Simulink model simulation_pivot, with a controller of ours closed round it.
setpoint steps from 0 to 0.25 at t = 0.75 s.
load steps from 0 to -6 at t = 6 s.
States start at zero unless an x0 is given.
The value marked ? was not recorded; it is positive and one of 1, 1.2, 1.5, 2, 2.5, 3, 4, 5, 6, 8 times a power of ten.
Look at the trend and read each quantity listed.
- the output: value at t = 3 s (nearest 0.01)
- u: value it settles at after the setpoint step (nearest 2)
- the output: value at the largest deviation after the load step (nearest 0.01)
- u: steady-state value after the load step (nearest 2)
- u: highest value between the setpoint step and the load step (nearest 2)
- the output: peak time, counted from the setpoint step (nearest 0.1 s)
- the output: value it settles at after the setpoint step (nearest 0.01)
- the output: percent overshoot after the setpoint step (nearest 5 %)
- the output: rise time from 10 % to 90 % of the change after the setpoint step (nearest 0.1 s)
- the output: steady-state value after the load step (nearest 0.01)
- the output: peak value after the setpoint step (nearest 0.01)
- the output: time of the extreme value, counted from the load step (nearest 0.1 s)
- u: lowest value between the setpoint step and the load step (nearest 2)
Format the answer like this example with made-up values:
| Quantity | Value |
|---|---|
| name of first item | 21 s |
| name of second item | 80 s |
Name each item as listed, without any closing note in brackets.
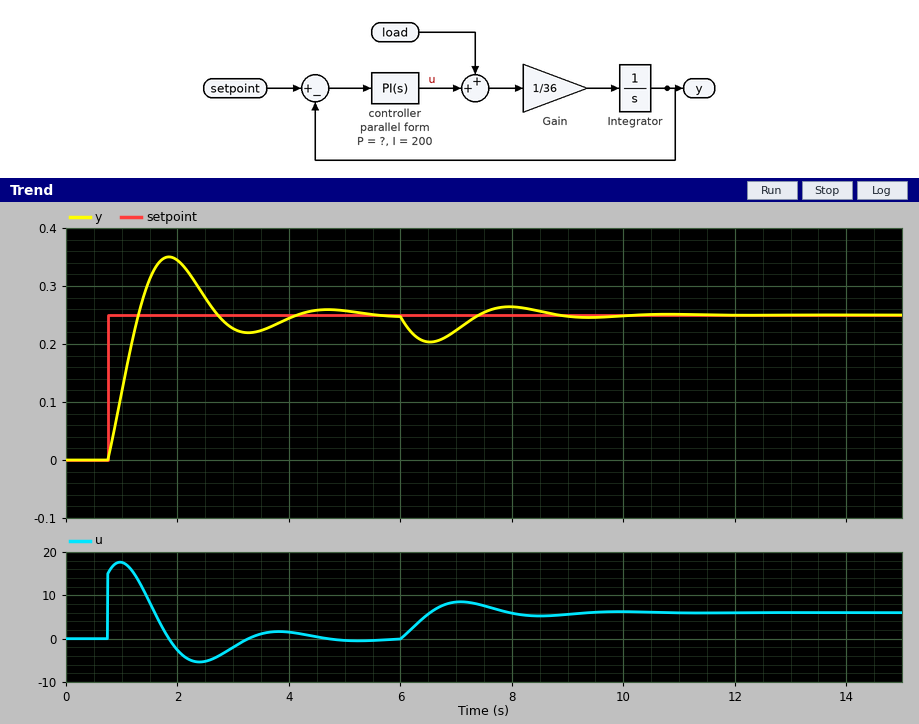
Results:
| Quantity | Value |
|---|---|
| the output: value at t = 3 s | 0.23 |
| u: value it settles at after the setpoint step | 0 |
| the output: value at the largest deviation after the load step | 0.20 |
| u: steady-state value after the load step | 6 |
| u: highest value between the setpoint step and the load step | 18 |
| the output: peak time, counted from the setpoint step | 1.1 s |
| the output: value it settles at after the setpoint step | 0.25 |
| the output: percent overshoot after the setpoint step | 40 % |
| the output: rise time from 10 % to 90 % of the change after the setpoint step | 0.4 s |
| the output: steady-state value after the load step | 0.25 |
| the output: peak value after the setpoint step | 0.35 |
| the output: time of the extreme value, counted from the load step | 0.5 s |
| u: lowest value between the setpoint step and the load step | -6 |
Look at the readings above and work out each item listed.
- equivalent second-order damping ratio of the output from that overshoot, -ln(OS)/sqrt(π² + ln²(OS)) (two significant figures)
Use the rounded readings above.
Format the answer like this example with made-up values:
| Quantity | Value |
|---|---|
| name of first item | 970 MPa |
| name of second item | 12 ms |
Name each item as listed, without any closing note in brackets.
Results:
| Quantity | Value |
|---|---|
| equivalent second-order damping ratio of the output from that overshoot, -ln(OS)/sqrt(π² + ln²(OS)) | 0.28 |
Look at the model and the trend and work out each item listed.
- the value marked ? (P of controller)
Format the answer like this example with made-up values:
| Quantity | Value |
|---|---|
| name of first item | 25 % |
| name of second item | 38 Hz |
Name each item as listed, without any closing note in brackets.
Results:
| Quantity | Value |
|---|---|
| the value marked ? | 60 |
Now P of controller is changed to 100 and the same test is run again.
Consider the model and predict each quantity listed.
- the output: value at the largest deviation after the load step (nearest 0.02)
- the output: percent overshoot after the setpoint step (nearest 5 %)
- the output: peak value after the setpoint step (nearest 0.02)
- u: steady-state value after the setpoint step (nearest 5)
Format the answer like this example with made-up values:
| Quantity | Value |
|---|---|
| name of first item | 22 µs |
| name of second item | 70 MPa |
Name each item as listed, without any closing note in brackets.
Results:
| Quantity | Value |
|---|---|
| the output: value at the largest deviation after the load step | 0.22 |
| the output: percent overshoot after the setpoint step | 25 % |
| the output: peak value after the setpoint step | 0.32 |
| u: steady-state value after the setpoint step | 0 |
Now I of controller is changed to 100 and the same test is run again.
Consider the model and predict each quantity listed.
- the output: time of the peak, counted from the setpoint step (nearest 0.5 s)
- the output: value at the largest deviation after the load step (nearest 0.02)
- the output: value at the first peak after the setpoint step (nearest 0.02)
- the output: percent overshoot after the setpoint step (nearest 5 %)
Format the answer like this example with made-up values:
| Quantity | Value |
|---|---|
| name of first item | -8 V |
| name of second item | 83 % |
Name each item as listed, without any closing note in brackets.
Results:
| Quantity | Value |
|---|---|
| the output: time of the peak, counted from the setpoint step | 1.5 s |
| the output: value at the largest deviation after the load step | 0.20 |
| the output: value at the first peak after the setpoint step | 0.32 |
| the output: percent overshoot after the setpoint step | 30 % |
